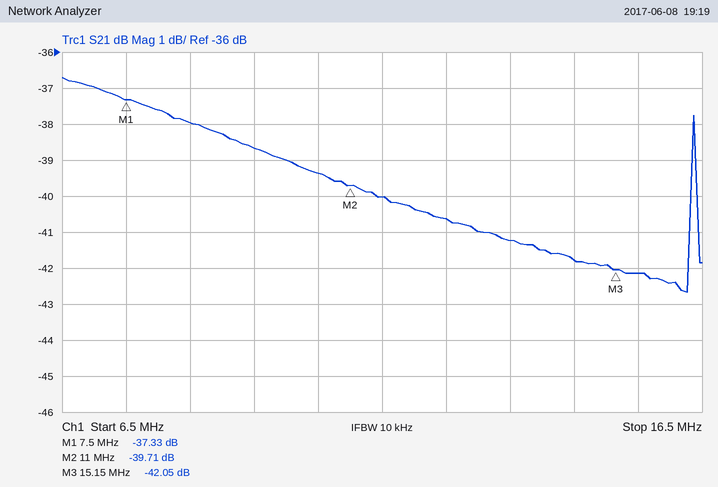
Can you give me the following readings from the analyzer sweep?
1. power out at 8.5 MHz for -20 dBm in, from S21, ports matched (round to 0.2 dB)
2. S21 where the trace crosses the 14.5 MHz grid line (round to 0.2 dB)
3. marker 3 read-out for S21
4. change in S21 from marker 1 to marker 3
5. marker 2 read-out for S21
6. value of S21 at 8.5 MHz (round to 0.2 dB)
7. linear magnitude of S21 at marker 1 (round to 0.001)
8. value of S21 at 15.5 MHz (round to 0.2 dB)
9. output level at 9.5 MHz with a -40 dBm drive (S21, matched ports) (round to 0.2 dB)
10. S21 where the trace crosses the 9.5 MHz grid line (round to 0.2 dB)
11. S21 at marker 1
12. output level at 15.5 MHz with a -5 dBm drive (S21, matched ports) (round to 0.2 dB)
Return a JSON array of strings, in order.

["-58.0 dBm", "-41.8 dB", "-42.05 dB", "-4.72 dB", "-39.71 dB", "-38.0 dB", "0.014", "-42.2 dB", "-78.6 dBm", "-38.6 dB", "-37.33 dB", "-47.2 dBm"]
